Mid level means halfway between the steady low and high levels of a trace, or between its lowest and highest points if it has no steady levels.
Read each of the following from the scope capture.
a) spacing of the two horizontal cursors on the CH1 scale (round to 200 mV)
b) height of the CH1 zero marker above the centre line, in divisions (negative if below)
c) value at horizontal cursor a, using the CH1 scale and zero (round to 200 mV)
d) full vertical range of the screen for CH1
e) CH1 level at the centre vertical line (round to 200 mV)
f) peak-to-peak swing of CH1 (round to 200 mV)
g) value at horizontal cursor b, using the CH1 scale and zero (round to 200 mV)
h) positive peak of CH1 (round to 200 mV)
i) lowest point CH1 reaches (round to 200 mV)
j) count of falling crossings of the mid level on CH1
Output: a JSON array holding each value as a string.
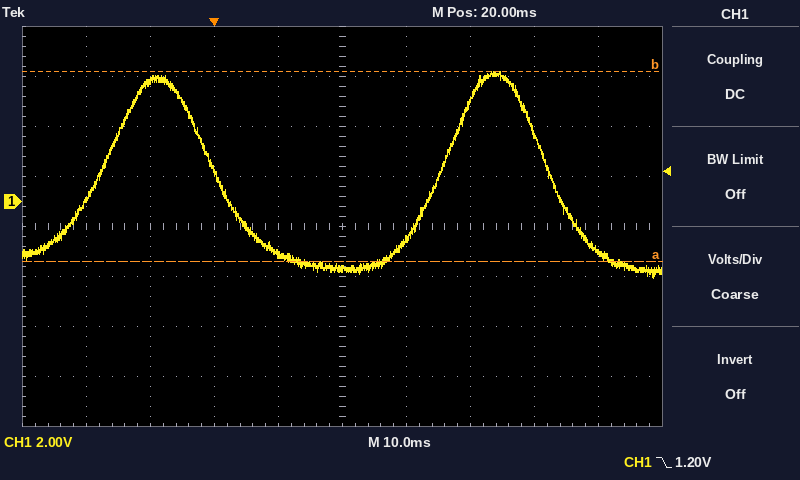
["7.6 V", "+0.5 div", "-2.4 V", "16 V", "-2.6 V", "8.2 V", "5.2 V", "5.2 V", "-3.0 V", "2"]
